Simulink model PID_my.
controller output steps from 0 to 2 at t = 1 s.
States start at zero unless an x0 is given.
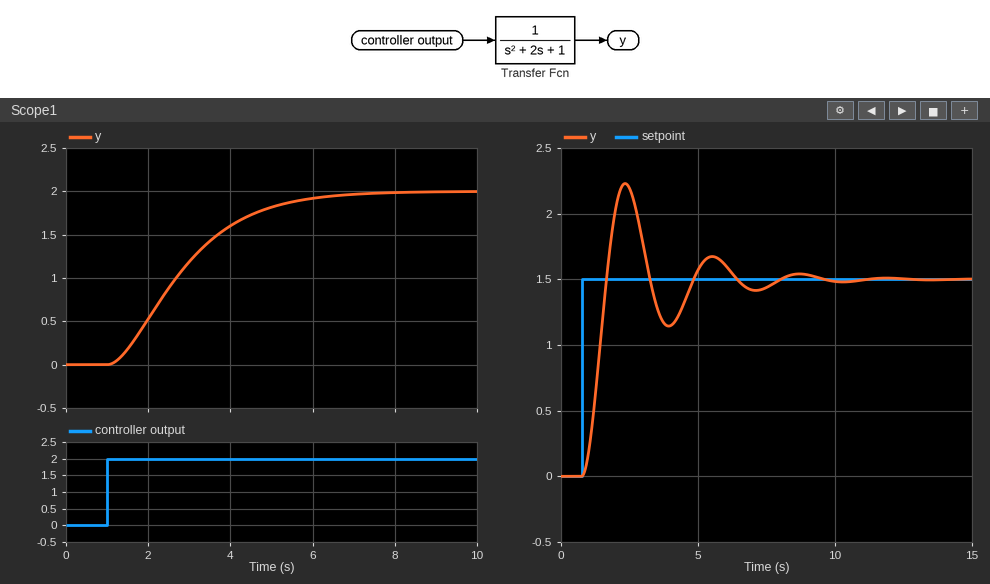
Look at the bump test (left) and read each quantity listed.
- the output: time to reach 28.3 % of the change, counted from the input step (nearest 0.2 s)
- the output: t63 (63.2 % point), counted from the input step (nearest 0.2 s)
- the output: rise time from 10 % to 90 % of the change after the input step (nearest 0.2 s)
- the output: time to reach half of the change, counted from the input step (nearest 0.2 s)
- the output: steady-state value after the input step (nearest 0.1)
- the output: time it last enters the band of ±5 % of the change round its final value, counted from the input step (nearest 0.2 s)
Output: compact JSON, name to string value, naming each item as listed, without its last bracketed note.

{"the output: time to reach 28.3 % of the change, counted from the input step": "1.0 s", "the output: t63 (63.2 % point), counted from the input step": "2.2 s", "the output: rise time from 10 % to 90 % of the change after the input step": "3.4 s", "the output: time to reach half of the change, counted from the input step": "1.6 s", "the output: steady-state value after the input step": "2.0", "the output: time it last enters the band of ±5 % of the change round its final value, counted from the input step": "4.8 s"}
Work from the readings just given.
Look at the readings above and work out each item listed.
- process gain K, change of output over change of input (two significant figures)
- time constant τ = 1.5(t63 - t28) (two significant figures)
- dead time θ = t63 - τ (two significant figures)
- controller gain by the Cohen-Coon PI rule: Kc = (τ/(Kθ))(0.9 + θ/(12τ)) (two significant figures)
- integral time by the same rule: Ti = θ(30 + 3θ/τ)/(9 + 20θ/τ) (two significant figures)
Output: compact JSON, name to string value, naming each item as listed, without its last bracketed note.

{"process gain K, change of output over change of input": "1.0", "time constant τ = 1.5(t63 - t28)": "1.8 s", "dead time θ = t63 - τ": "0.40 s", "controller gain by the Cohen-Coon PI rule: Kc = (τ/(Kθ))(0.9 + θ/(12τ))": "4.1", "integral time by the same rule: Ti = θ(30 + 3θ/τ)/(9 + 20θ/τ)": "0.91 s"}
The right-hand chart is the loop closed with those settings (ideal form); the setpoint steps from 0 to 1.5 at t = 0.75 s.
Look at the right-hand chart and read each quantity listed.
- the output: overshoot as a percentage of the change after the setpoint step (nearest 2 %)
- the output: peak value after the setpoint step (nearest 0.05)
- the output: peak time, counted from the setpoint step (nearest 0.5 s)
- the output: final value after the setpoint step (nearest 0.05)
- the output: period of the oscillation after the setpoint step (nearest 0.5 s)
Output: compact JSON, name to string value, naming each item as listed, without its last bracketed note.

{"the output: overshoot as a percentage of the change after the setpoint step": "48 %", "the output: peak value after the setpoint step": "2.25", "the output: peak time, counted from the setpoint step": "1.5 s", "the output: final value after the setpoint step": "1.50", "the output: period of the oscillation after the setpoint step": "3.0 s"}
